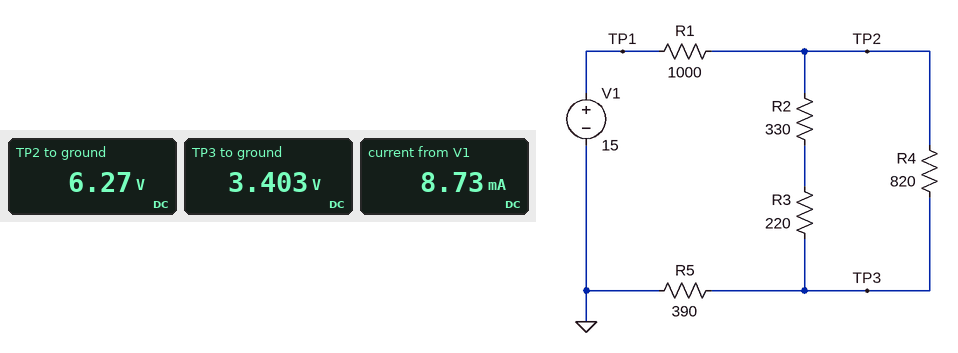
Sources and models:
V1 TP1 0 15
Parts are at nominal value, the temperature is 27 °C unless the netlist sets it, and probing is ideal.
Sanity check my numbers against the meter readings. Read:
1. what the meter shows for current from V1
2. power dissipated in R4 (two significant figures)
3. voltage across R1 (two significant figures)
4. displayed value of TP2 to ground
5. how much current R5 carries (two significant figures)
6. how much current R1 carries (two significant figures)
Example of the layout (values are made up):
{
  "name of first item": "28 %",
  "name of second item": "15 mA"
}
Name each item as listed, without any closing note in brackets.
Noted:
{
  "what the meter shows for current from V1": "8.73 mA",
  "power dissipated in R4": "10 mW",
  "voltage across R1": "8.7 V",
  "displayed value of TP2 to ground": "6.27 V",
  "how much current R5 carries": "8.7 mA",
  "how much current R1 carries": "8.7 mA"
}
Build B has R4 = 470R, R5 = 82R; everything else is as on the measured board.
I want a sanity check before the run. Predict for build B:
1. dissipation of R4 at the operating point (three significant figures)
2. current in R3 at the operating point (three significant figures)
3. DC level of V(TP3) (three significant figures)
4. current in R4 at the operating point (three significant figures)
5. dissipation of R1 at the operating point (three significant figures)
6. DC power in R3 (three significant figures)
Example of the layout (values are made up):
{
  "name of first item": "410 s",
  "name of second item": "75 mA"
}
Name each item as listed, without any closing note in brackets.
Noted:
{
  "dissipation of R4 at the operating point": "17.2 mW",
  "current in R3 at the operating point": "5.18 mA",
  "DC level of V(TP3)": "921 mV",
  "current in R4 at the operating point": "6.06 mA",
  "dissipation of R1 at the operating point": "126 mW",
  "DC power in R3": "5.89 mW"
}
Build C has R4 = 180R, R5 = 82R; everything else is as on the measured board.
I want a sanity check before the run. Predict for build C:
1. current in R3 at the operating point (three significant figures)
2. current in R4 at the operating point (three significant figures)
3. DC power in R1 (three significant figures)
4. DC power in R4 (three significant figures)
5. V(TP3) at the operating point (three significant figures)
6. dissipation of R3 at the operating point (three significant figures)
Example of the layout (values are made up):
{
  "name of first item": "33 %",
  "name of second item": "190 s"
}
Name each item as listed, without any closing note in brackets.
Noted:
{
  "current in R3 at the operating point": "3.04 mA",
  "current in R4 at the operating point": "9.28 mA",
  "DC power in R1": "152 mW",
  "DC power in R4": "15.5 mW",
  "V(TP3) at the operating point": "1.01 V",
  "dissipation of R3 at the operating point": "2.03 mW"
}
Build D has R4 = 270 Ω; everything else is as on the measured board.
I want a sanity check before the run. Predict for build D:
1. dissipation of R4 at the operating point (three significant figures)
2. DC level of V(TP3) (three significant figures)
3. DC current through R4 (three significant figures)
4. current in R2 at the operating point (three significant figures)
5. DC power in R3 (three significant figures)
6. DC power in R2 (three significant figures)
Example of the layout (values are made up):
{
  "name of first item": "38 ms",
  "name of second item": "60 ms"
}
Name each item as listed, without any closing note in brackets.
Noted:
{
  "dissipation of R4 at the operating point": "11.1 mW",
  "DC level of V(TP3)": "3.72 V",
  "DC current through R4": "6.40 mA",
  "current in R2 at the operating point": "3.14 mA",
  "DC power in R3": "2.17 mW",
  "DC power in R2": "3.26 mW"
}
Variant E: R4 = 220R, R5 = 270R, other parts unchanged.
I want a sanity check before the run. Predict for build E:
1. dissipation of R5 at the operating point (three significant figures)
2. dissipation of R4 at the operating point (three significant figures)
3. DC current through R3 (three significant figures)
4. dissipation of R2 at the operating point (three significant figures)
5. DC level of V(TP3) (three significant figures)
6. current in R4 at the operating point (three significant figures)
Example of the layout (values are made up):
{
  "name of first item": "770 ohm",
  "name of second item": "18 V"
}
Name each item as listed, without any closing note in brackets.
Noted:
{
  "dissipation of R5 at the operating point": "29.8 mW",
  "dissipation of R4 at the operating point": "12.4 mW",
  "DC current through R3": "3.00 mA",
  "dissipation of R2 at the operating point": "2.98 mW",
  "DC level of V(TP3)": "2.84 V",
  "current in R4 at the operating point": "7.51 mA"
}
